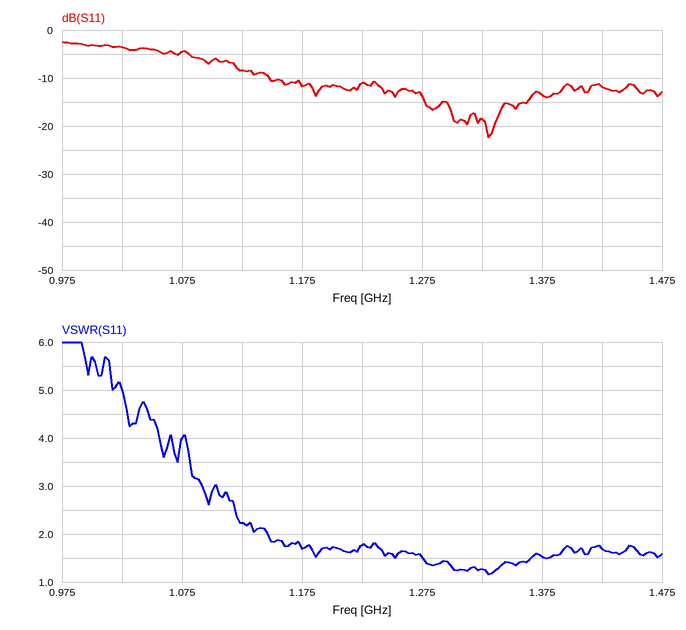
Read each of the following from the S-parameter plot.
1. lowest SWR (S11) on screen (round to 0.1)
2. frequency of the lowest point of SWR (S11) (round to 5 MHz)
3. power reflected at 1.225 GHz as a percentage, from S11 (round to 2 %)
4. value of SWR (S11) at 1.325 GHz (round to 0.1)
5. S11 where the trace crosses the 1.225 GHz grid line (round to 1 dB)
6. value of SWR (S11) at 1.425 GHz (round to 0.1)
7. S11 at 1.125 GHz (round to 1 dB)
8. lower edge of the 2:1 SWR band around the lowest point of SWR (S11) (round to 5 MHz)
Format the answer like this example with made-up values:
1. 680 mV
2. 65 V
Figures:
1. 1.2
2. 1.330 GHz
3. 8 %
4. 1.3
5. -11 dB
6. 1.7
7. -8 dB
8. 1.145 GHz
